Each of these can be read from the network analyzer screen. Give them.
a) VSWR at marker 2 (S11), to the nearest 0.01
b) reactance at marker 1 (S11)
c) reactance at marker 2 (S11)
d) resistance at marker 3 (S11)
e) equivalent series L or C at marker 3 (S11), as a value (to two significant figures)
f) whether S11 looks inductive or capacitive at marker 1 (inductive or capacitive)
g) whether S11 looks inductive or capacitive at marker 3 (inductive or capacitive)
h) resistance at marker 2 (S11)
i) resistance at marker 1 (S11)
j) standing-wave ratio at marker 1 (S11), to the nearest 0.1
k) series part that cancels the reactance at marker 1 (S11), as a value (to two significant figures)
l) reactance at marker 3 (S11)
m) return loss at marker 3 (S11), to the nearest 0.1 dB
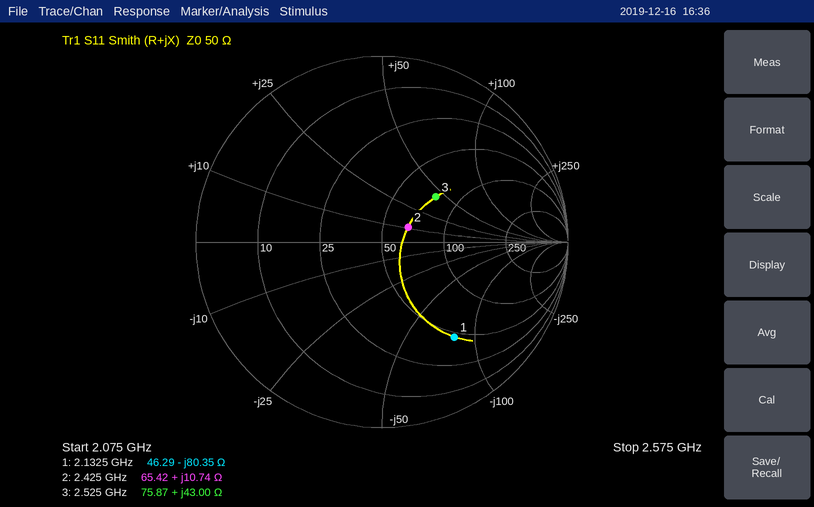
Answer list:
1.39
-80.35 Ω
+10.74 Ω
75.87 Ω
2.7 nH
capacitive
inductive
65.42 Ω
46.29 Ω
4.6
6.0 nH
+43.00 Ω
8.5 dB
